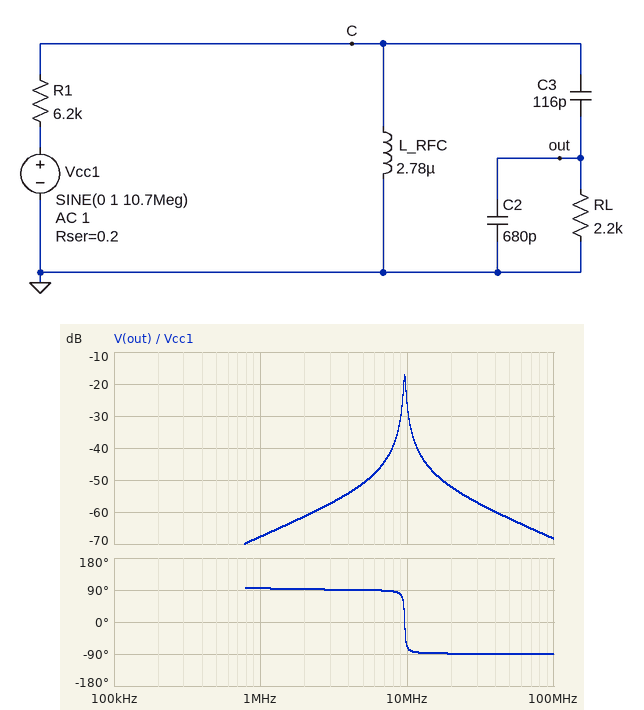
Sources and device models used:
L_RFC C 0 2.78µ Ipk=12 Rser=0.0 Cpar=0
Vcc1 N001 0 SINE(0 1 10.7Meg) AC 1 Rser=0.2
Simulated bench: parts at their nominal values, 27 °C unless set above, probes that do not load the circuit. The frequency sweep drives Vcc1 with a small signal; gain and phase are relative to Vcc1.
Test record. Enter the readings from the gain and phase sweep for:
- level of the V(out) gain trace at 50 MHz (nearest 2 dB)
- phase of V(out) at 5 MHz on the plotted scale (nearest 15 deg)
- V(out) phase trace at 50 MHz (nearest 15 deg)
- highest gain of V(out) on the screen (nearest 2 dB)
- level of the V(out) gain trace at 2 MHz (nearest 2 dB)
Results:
-62 dB
90 deg
-90 deg
-18 dB
-62 dB
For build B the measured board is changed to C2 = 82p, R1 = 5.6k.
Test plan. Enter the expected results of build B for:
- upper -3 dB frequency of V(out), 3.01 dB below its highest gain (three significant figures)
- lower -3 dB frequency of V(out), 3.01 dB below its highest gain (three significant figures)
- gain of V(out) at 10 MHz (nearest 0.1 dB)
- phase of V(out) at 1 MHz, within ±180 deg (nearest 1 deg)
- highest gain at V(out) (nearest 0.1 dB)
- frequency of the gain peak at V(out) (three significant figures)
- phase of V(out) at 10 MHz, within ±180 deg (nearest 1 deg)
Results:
14.3 MHz
13.2 MHz
-28.3 dB
110 deg
-10.1 dB
13.8 MHz
85 deg
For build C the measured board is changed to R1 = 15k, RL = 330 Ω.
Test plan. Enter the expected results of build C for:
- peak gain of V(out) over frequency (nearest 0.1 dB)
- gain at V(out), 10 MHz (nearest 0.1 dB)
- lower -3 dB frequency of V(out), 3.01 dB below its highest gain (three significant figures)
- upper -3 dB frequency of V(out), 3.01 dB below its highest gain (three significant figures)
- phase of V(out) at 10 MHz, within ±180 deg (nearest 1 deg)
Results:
-22.6 dB
-34.6 dB
9.48 MHz
9.69 MHz
-72 deg
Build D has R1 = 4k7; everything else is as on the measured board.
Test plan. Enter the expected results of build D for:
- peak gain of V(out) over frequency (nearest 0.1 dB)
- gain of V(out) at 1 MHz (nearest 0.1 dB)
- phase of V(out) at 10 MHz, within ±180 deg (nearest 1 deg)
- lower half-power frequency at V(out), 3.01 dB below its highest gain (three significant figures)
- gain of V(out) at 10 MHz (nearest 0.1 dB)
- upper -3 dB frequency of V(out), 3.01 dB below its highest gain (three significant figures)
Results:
-17.1 dB
-65.3 dB
-66 deg
9.41 MHz
-25.0 dB
9.77 MHz
